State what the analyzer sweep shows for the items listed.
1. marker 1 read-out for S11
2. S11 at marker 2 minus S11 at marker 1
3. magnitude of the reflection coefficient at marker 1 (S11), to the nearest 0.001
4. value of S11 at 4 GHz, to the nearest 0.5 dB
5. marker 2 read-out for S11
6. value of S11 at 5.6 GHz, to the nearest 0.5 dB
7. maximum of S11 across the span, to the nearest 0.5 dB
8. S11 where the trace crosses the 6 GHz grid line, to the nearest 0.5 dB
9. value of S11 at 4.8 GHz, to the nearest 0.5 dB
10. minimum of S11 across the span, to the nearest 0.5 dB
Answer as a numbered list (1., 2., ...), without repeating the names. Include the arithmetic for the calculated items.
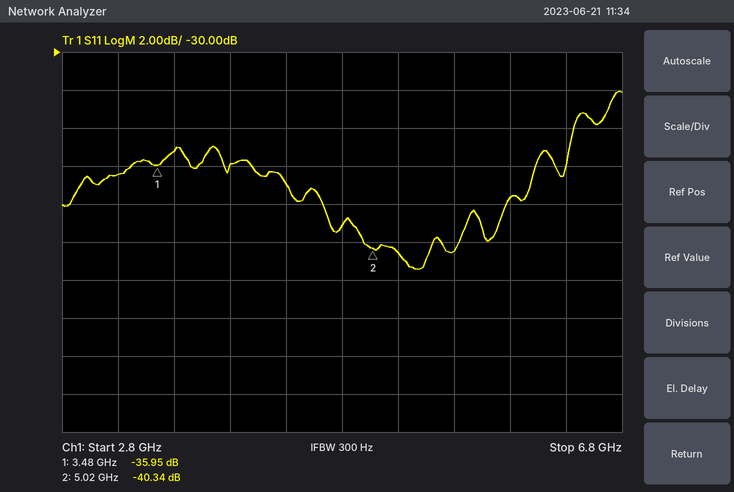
1. -35.95 dB
2. -40.34 − (-35.95) = -4.39 dB
3. 10^(-35.95/20) ≈ 0.016
4. -36.0 dB
5. -40.34 dB
6. -40.5 dB
7. -32.0 dB
8. -37.5 dB
9. -39.0 dB
10. -41.5 dB
